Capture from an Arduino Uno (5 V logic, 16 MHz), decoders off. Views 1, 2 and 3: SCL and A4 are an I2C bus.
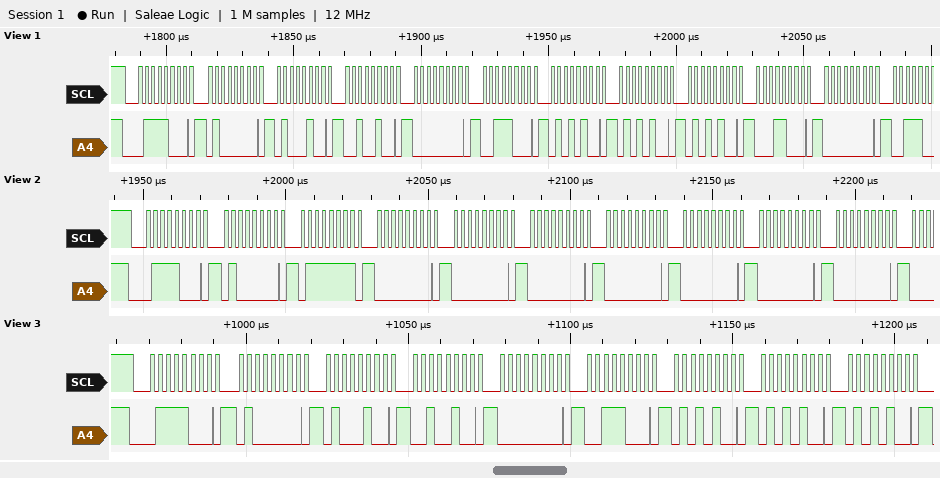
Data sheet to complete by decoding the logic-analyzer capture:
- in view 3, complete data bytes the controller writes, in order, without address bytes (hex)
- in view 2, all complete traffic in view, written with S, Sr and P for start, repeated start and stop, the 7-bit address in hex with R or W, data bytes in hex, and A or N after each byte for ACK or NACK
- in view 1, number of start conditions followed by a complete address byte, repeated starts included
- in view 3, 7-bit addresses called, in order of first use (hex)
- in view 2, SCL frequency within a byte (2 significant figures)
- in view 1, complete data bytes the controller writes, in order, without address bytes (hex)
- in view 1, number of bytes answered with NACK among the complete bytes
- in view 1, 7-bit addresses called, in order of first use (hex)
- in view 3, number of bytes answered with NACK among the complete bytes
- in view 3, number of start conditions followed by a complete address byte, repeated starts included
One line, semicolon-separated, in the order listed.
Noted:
40 44 24 00 38 54 54 54; S 3CW A 40 A 7F A 00 A 00 A 00 A 00 A 00 A 00 A 00 A; 1; 0x3C; 400 kHz; 40 44 24 00 38 54 54 54 18 00; 0; 0x3C; 0; 1
